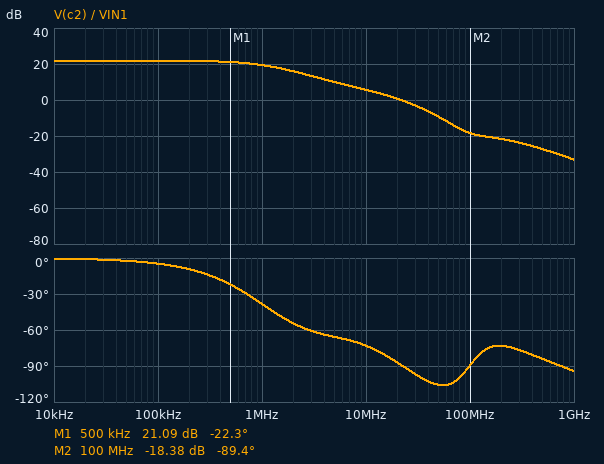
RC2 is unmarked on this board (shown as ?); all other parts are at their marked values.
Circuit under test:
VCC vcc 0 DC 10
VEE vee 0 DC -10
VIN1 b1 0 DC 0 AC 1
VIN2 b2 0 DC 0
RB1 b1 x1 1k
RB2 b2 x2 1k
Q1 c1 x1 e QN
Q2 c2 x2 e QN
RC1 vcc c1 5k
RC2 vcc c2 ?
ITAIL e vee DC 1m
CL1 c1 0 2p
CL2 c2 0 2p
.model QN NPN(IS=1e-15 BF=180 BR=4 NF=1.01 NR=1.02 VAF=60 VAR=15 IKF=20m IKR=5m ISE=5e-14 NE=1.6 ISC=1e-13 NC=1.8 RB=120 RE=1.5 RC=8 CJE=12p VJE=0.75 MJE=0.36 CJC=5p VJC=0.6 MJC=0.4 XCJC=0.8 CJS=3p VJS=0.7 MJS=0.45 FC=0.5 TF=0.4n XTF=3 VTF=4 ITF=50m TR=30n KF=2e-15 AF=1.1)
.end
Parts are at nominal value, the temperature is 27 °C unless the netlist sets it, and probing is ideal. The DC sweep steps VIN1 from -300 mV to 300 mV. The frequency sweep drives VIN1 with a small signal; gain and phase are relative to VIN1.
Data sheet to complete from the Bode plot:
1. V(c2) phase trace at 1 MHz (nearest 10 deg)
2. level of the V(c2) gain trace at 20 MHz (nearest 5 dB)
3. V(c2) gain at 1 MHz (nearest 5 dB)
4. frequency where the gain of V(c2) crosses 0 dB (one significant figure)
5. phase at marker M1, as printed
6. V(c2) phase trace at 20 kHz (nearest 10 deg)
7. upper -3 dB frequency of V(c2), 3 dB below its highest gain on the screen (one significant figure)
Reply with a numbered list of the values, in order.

1. -40 deg
2. 0 dB
3. 20 dB
4. 20 MHz
5. -22.3 deg
6. 0 deg
7. 1 MHz
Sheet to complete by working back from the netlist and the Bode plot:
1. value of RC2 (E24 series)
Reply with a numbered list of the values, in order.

1. 1.6 kΩ
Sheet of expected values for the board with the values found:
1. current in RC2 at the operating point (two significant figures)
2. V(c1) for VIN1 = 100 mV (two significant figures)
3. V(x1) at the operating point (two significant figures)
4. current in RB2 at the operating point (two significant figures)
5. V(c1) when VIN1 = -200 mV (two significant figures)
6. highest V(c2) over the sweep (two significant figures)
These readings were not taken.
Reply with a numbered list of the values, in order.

1. 500 µA
2. 5.2 V
3. -3.7 mV
4. 3.7 µA
5. 10 V
6. 10 V
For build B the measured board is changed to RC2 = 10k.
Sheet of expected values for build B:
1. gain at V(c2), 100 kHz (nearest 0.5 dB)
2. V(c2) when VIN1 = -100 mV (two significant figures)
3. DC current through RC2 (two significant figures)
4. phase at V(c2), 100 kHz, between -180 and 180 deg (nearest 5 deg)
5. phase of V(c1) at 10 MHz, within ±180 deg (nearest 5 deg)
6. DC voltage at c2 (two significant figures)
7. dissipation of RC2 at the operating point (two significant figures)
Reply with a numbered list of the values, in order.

1. 37.5 dB
2. 450 mV
3. 490 µA
4. -10 deg
5. 85 deg
6. 5.1 V
7. 2.4 mW
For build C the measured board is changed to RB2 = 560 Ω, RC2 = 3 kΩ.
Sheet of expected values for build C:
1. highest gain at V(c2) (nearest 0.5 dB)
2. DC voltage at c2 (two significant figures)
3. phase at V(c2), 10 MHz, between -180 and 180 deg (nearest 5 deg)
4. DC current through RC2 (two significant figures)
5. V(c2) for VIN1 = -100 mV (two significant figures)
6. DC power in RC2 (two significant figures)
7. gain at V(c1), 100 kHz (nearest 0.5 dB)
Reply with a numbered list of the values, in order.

1. 27.5 dB
2. 8.5 V
3. -85 deg
4. 510 µA
5. 7.1 V
6. 790 µW
7. 32.0 dB
